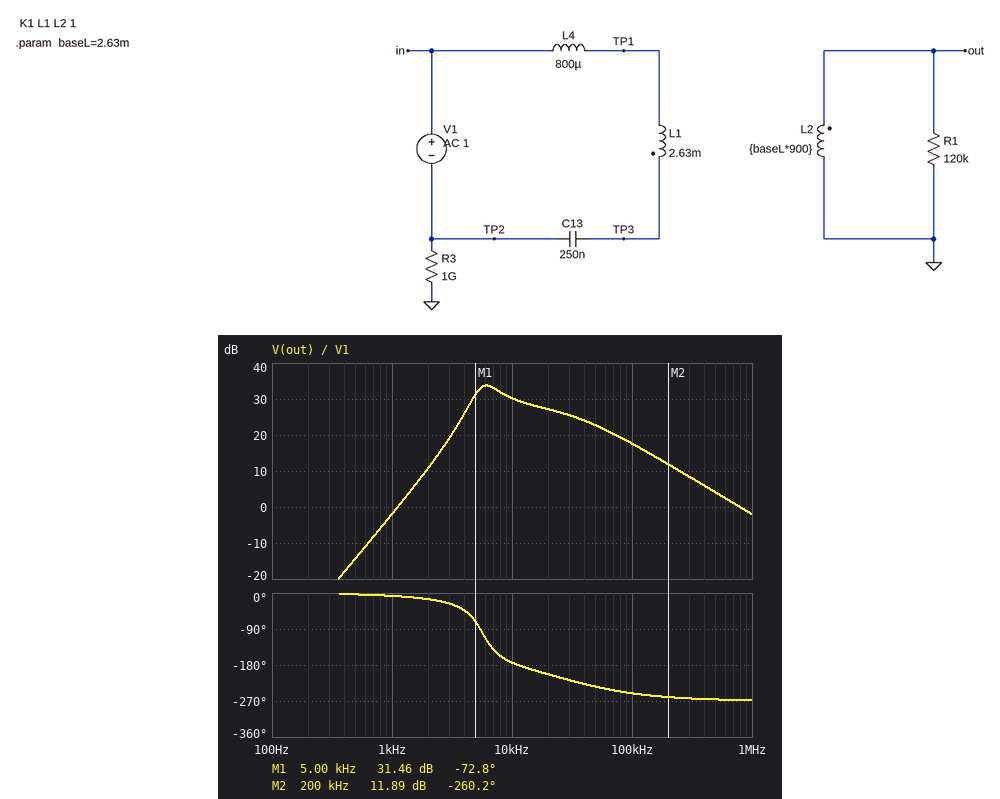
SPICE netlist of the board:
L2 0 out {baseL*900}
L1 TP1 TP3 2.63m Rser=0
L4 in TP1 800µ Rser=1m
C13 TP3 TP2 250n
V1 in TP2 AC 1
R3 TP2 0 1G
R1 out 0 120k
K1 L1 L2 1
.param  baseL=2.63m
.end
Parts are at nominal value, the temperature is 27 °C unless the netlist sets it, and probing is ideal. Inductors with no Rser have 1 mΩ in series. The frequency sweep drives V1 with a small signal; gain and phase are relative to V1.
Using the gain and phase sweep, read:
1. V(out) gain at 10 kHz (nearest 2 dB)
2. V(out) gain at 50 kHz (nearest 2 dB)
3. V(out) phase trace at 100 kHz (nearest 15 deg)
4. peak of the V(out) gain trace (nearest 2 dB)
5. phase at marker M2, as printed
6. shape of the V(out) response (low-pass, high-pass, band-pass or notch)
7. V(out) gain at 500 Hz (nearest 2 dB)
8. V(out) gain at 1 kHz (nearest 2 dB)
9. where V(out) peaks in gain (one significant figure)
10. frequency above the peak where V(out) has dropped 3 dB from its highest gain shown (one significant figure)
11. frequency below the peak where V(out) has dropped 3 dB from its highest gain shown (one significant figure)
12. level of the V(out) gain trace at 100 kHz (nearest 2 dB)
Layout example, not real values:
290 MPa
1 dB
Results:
30 dB
22 dB
-255 deg
34 dB
-260.2 deg
band-pass
-14 dB
-2 dB
6 kHz
9 kHz
5 kHz
18 dB
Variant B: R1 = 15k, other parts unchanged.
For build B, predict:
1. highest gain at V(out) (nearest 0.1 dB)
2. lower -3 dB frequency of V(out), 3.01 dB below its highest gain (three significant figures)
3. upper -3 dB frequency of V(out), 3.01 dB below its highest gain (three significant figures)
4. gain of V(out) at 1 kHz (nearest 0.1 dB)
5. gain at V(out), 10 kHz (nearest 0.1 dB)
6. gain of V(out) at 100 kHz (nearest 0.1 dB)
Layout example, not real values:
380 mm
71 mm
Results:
29.6 dB
9.58 kHz
12.9 kHz
-5.0 dB
27.8 dB
0.1 dB
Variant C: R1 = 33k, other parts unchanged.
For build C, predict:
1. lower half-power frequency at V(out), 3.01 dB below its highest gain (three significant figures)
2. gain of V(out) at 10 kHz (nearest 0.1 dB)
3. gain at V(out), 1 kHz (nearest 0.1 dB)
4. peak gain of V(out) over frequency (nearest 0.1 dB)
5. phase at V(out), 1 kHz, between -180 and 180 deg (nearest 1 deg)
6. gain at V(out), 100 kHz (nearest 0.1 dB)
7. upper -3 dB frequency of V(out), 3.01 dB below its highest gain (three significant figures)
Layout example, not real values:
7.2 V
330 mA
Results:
7.64 kHz
29.6 dB
-2.7 dB
29.7 dB
-25 deg
6.9 dB
14.6 kHz
